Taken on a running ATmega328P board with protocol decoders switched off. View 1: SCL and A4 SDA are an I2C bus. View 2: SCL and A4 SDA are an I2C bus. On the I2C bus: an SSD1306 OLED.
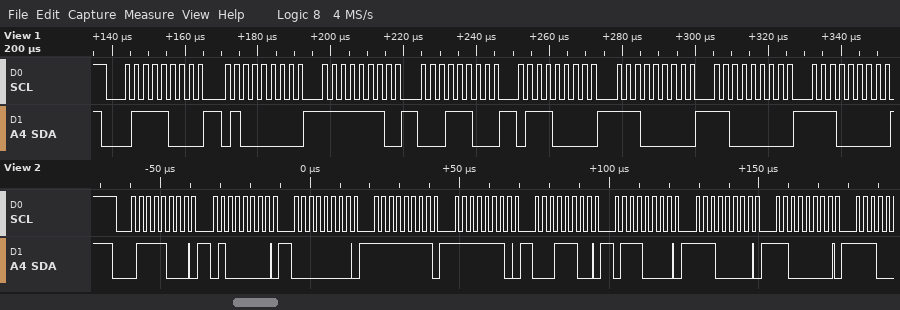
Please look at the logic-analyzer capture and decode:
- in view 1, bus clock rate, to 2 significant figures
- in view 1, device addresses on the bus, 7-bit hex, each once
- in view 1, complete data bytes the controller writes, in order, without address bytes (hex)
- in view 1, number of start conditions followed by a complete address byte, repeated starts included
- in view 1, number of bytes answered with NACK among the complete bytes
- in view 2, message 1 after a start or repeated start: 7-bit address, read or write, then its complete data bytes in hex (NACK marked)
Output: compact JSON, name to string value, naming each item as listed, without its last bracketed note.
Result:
{"in view 1, bus clock rate, to 2 significant figures": "400 kHz", "in view 1, device addresses on the bus, 7-bit hex, each once": "0x3C", "in view 1, complete data bytes the controller writes, in order, without address bytes": "40 FE 1C 70 E0 C0 E0", "in view 1, number of start conditions followed by a complete address byte, repeated starts included": "1", "in view 1, number of bytes answered with NACK among the complete bytes": "0", "in view 2, message 1 after a start or repeated start: 7-bit address, read or write, then its complete data bytes in hex": "0x3C write: 40 00 FF FE 1C 70 E0 C0"}
